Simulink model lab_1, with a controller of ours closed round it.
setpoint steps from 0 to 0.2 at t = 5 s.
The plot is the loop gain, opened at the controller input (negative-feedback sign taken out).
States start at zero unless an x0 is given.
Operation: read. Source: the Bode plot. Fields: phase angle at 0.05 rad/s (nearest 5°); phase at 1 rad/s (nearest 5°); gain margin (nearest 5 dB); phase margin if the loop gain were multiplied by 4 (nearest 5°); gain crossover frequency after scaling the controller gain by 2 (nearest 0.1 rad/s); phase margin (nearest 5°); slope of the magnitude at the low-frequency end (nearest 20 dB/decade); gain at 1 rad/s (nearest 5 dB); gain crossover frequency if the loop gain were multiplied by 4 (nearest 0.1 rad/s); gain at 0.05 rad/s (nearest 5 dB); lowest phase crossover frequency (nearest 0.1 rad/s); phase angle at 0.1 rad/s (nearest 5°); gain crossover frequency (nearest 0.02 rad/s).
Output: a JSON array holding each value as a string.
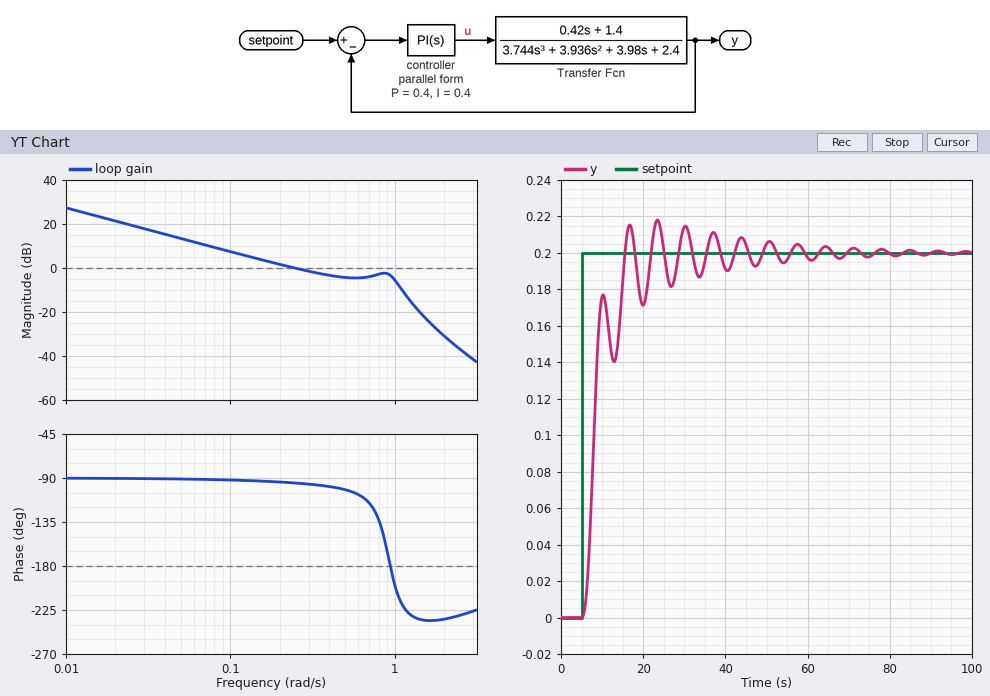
["-90°", "-200°", "5 dB", "-45°", "1.0 rad/s", "85°", "-20 dB/decade", "-5 dB", "1.2 rad/s", "15 dB", "0.9 rad/s", "-90°", "0.24 rad/s"]
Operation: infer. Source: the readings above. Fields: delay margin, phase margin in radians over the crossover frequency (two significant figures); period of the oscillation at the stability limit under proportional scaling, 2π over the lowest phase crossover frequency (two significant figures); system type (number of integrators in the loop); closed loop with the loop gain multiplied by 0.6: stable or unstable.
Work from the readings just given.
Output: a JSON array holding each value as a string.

["6.2 s", "7.0 s", "1", "stable"]
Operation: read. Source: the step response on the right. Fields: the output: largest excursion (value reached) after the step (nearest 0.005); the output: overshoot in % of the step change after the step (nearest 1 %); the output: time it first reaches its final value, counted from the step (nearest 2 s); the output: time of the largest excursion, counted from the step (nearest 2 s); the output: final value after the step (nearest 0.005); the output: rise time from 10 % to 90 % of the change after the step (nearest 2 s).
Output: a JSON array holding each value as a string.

["0.220", "9 %", "10 s", "18 s", "0.200", "8 s"]
